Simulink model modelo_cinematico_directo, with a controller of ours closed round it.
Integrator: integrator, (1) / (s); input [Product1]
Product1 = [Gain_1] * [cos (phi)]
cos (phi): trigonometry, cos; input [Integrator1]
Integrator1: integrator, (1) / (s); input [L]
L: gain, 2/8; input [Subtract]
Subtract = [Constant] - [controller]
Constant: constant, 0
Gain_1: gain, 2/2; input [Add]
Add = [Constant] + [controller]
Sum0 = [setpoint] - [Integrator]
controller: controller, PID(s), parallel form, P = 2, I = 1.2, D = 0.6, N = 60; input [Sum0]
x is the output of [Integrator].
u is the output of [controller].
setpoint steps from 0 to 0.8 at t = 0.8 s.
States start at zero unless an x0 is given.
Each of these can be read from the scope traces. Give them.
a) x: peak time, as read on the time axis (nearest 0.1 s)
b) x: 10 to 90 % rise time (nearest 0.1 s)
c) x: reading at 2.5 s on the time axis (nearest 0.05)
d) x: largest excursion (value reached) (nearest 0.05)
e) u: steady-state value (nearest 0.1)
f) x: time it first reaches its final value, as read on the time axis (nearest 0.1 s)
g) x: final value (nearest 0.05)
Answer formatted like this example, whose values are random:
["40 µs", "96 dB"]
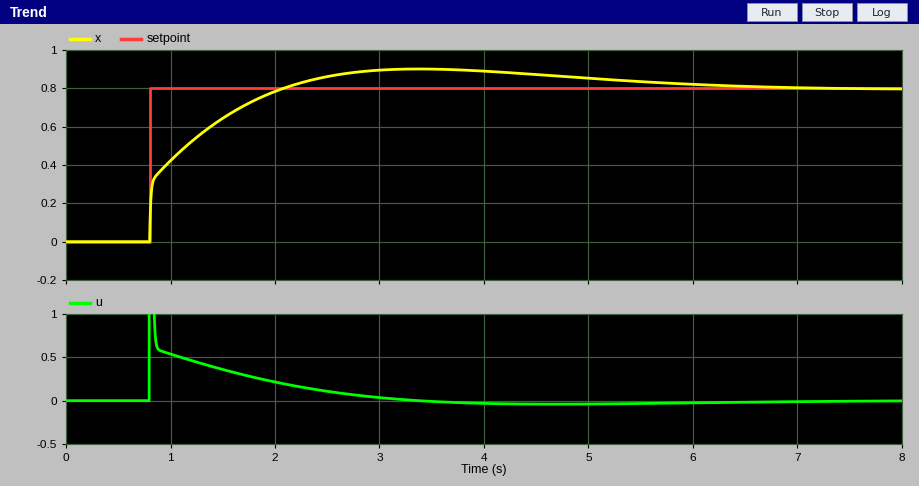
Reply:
["3.4 s", "0.9 s", "0.85", "0.90", "0.0", "2.1 s", "0.80"]
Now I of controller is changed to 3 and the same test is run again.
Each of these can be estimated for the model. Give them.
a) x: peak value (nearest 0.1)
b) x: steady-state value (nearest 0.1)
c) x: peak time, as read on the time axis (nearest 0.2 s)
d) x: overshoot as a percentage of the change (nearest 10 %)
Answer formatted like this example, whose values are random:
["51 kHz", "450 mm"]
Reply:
["1.0", "0.8", "2.6 s", "20 %"]
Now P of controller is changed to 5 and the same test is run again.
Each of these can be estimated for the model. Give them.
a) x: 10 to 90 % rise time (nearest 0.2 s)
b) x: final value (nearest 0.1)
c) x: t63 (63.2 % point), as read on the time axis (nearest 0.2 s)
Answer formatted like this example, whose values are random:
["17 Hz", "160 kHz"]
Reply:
["0.6 s", "0.8", "1.0 s"]
